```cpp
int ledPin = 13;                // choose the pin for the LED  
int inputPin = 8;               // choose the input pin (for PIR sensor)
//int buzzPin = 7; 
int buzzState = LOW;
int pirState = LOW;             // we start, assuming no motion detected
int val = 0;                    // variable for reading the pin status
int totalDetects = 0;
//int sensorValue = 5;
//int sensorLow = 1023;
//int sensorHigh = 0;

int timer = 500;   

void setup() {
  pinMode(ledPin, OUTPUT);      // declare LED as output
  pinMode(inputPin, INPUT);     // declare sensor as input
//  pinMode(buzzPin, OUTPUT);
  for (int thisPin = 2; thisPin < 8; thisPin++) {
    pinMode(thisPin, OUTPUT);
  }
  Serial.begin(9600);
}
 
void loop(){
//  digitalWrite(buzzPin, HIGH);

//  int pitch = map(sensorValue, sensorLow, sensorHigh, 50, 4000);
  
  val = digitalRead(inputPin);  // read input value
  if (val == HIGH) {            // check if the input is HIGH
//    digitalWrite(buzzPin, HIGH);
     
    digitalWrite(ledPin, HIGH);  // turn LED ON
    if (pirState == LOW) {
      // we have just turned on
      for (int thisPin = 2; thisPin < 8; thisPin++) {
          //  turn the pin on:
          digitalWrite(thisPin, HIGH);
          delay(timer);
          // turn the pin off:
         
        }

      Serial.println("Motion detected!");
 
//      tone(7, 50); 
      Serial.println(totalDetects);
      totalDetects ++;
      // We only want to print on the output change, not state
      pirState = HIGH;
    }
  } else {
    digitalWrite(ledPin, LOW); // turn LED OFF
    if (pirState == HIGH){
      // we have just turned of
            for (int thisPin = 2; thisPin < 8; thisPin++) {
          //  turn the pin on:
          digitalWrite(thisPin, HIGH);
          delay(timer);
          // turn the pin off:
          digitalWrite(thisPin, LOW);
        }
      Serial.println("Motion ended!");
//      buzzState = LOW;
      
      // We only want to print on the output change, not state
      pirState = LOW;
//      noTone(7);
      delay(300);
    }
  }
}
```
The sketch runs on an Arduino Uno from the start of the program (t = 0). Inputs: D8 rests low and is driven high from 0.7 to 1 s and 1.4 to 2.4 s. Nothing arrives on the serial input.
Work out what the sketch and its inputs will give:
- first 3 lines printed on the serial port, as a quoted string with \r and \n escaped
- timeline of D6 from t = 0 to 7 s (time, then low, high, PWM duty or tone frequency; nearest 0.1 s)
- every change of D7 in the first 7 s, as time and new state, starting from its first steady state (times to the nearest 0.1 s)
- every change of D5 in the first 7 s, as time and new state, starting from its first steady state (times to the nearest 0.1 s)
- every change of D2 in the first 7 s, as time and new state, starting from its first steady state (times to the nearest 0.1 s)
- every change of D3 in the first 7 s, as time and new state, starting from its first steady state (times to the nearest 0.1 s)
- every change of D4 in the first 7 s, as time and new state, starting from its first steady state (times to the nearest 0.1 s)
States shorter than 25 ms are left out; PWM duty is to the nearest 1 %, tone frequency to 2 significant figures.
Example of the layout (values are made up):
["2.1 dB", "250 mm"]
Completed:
["\"Motion detected!\\r\\n0\\r\\nMotion ended!\\r\\n\"", "0 s low; 2.7 s high; 6.2 s low", "0 s low; 3.2 s high; 6.7 s low", "0 s low; 2.2 s high; 5.7 s low", "0 s low; 0.7 s high; 4.2 s low", "0 s low; 1.2 s high; 4.7 s low", "0 s low; 1.7 s high; 5.2 s low"]
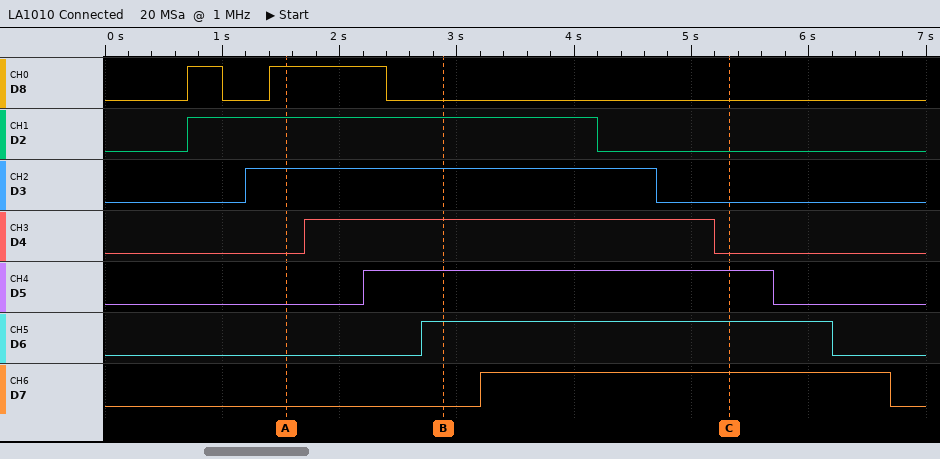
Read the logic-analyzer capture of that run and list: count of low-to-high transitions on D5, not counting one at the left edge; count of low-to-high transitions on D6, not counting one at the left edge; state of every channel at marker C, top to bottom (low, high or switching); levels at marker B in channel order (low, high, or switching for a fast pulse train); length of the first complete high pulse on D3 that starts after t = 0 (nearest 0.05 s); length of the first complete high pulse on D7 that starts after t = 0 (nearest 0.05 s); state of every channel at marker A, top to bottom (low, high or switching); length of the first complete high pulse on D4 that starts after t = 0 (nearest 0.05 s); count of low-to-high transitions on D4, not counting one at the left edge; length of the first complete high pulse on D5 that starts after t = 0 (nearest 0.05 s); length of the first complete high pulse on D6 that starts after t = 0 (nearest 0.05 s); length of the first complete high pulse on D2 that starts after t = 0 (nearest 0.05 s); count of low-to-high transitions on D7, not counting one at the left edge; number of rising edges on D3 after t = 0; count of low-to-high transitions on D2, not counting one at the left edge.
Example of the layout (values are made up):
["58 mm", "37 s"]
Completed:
["1", "1", "D8 low, D2 low, D3 low, D4 low, D5 high, D6 high, D7 high", "D8 low, D2 high, D3 high, D4 high, D5 high, D6 high, D7 low", "3.50 s", "3.50 s", "D8 high, D2 high, D3 high, D4 low, D5 low, D6 low, D7 low", "3.50 s", "1", "3.50 s", "3.50 s", "3.50 s", "1", "1", "1"]
